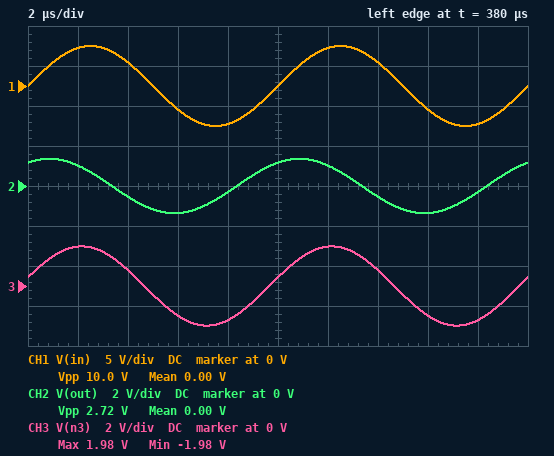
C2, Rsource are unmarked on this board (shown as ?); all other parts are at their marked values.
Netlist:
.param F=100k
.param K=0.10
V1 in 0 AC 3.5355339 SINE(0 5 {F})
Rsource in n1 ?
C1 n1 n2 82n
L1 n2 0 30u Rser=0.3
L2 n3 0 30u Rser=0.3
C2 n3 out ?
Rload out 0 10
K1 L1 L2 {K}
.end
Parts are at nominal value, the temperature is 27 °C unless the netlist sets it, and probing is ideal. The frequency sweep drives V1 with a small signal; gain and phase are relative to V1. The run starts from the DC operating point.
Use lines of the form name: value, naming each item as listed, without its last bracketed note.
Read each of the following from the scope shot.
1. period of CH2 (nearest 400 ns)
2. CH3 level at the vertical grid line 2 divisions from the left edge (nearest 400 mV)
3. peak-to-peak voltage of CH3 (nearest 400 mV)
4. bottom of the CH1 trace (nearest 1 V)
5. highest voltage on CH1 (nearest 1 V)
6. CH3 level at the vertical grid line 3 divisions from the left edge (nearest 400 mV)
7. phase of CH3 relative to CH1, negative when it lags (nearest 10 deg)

period of CH2: 10.0 µs
CH3 level at the vertical grid line 2 divisions from the left edge: 800 mV
peak-to-peak voltage of CH3: 4.0 V
bottom of the CH1 trace: -5 V
highest voltage on CH1: 5 V
CH3 level at the vertical grid line 3 divisions from the left edge: -1.6 V
phase of CH3 relative to CH1, negative when it lags: 10 deg
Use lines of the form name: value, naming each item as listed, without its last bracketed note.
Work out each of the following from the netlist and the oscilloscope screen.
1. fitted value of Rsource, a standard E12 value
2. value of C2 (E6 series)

fitted value of Rsource, a standard E12 value: 4.7 Ω
value of C2: 150 nF
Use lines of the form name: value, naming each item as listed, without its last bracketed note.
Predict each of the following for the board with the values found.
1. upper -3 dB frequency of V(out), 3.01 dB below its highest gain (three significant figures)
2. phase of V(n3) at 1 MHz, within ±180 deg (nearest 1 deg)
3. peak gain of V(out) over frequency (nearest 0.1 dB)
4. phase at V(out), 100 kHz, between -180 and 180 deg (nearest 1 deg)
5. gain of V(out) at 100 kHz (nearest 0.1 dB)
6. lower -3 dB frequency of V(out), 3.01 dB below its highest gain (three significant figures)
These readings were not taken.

upper -3 dB frequency of V(out), 3.01 dB below its highest gain: 115 kHz
phase of V(n3) at 1 MHz, within ±180 deg: -91 deg
peak gain of V(out) over frequency: -11.3 dB
phase at V(out), 100 kHz, between -180 and 180 deg: 59 deg
gain of V(out) at 100 kHz: -11.3 dB
lower -3 dB frequency of V(out), 3.01 dB below its highest gain: 88.0 kHz
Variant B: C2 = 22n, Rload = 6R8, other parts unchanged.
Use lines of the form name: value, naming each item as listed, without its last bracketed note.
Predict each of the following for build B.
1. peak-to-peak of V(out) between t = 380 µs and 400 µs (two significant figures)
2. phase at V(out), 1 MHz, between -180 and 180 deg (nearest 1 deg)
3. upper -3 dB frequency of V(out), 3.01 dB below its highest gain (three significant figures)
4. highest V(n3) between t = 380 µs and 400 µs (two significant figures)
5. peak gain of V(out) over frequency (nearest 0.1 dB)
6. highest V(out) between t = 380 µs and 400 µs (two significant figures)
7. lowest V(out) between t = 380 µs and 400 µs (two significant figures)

peak-to-peak of V(out) between t = 380 µs and 400 µs: 470 mV
phase at V(out), 1 MHz, between -180 and 180 deg: -86 deg
upper -3 dB frequency of V(out), 3.01 dB below its highest gain: 215 kHz
highest V(n3) between t = 380 µs and 400 µs: 2.5 V
peak gain of V(out) over frequency: -17.9 dB
highest V(out) between t = 380 µs and 400 µs: 240 mV
lowest V(out) between t = 380 µs and 400 µs: -240 mV
